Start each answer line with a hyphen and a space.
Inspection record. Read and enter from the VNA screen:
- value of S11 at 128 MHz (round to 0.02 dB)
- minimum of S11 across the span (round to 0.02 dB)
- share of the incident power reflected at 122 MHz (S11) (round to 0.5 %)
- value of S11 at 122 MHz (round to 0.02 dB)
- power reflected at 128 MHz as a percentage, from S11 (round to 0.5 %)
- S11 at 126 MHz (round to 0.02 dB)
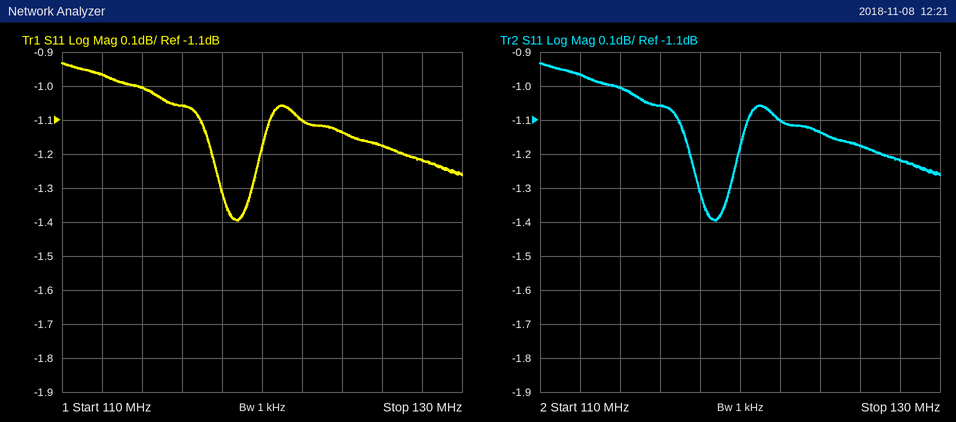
- -1.22 dB
- -1.40 dB
- 77.5 %
- -1.10 dB
- 75.5 %
- -1.18 dB
